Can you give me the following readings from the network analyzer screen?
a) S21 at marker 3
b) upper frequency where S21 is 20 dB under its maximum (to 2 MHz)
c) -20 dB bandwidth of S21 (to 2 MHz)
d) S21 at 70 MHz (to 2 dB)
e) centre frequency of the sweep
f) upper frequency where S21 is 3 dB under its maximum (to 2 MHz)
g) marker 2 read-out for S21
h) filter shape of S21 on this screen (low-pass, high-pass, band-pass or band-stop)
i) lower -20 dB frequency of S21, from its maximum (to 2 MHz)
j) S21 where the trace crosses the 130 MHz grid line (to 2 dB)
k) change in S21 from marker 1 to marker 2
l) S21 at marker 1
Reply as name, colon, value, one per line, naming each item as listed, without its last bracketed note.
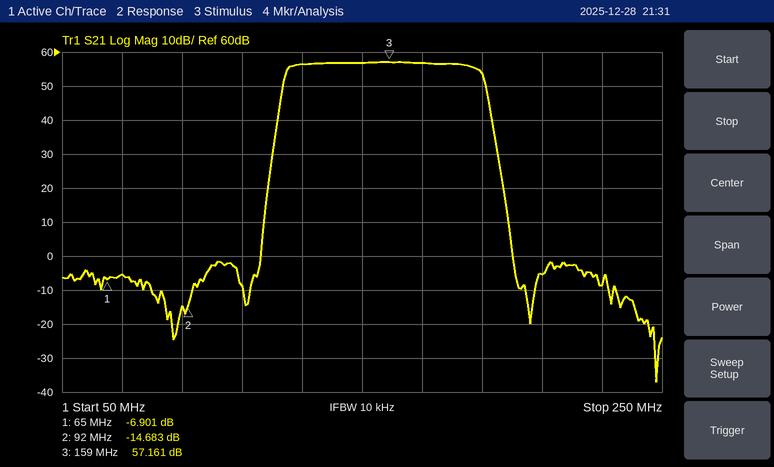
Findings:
S21 at marker 3: 57.161 dB
upper frequency where S21 is 20 dB under its maximum: 194 MHz
-20 dB bandwidth of S21: 72 MHz
S21 at 70 MHz: -6 dB
centre frequency of the sweep: 150 MHz
upper frequency where S21 is 3 dB under its maximum: 190 MHz
marker 2 read-out for S21: -14.683 dB
filter shape of S21 on this screen: band-pass
lower -20 dB frequency of S21, from its maximum: 122 MHz
S21 where the trace crosses the 130 MHz grid line: 56 dB
change in S21 from marker 1 to marker 2: -7.782 dB
S21 at marker 1: -6.901 dB
